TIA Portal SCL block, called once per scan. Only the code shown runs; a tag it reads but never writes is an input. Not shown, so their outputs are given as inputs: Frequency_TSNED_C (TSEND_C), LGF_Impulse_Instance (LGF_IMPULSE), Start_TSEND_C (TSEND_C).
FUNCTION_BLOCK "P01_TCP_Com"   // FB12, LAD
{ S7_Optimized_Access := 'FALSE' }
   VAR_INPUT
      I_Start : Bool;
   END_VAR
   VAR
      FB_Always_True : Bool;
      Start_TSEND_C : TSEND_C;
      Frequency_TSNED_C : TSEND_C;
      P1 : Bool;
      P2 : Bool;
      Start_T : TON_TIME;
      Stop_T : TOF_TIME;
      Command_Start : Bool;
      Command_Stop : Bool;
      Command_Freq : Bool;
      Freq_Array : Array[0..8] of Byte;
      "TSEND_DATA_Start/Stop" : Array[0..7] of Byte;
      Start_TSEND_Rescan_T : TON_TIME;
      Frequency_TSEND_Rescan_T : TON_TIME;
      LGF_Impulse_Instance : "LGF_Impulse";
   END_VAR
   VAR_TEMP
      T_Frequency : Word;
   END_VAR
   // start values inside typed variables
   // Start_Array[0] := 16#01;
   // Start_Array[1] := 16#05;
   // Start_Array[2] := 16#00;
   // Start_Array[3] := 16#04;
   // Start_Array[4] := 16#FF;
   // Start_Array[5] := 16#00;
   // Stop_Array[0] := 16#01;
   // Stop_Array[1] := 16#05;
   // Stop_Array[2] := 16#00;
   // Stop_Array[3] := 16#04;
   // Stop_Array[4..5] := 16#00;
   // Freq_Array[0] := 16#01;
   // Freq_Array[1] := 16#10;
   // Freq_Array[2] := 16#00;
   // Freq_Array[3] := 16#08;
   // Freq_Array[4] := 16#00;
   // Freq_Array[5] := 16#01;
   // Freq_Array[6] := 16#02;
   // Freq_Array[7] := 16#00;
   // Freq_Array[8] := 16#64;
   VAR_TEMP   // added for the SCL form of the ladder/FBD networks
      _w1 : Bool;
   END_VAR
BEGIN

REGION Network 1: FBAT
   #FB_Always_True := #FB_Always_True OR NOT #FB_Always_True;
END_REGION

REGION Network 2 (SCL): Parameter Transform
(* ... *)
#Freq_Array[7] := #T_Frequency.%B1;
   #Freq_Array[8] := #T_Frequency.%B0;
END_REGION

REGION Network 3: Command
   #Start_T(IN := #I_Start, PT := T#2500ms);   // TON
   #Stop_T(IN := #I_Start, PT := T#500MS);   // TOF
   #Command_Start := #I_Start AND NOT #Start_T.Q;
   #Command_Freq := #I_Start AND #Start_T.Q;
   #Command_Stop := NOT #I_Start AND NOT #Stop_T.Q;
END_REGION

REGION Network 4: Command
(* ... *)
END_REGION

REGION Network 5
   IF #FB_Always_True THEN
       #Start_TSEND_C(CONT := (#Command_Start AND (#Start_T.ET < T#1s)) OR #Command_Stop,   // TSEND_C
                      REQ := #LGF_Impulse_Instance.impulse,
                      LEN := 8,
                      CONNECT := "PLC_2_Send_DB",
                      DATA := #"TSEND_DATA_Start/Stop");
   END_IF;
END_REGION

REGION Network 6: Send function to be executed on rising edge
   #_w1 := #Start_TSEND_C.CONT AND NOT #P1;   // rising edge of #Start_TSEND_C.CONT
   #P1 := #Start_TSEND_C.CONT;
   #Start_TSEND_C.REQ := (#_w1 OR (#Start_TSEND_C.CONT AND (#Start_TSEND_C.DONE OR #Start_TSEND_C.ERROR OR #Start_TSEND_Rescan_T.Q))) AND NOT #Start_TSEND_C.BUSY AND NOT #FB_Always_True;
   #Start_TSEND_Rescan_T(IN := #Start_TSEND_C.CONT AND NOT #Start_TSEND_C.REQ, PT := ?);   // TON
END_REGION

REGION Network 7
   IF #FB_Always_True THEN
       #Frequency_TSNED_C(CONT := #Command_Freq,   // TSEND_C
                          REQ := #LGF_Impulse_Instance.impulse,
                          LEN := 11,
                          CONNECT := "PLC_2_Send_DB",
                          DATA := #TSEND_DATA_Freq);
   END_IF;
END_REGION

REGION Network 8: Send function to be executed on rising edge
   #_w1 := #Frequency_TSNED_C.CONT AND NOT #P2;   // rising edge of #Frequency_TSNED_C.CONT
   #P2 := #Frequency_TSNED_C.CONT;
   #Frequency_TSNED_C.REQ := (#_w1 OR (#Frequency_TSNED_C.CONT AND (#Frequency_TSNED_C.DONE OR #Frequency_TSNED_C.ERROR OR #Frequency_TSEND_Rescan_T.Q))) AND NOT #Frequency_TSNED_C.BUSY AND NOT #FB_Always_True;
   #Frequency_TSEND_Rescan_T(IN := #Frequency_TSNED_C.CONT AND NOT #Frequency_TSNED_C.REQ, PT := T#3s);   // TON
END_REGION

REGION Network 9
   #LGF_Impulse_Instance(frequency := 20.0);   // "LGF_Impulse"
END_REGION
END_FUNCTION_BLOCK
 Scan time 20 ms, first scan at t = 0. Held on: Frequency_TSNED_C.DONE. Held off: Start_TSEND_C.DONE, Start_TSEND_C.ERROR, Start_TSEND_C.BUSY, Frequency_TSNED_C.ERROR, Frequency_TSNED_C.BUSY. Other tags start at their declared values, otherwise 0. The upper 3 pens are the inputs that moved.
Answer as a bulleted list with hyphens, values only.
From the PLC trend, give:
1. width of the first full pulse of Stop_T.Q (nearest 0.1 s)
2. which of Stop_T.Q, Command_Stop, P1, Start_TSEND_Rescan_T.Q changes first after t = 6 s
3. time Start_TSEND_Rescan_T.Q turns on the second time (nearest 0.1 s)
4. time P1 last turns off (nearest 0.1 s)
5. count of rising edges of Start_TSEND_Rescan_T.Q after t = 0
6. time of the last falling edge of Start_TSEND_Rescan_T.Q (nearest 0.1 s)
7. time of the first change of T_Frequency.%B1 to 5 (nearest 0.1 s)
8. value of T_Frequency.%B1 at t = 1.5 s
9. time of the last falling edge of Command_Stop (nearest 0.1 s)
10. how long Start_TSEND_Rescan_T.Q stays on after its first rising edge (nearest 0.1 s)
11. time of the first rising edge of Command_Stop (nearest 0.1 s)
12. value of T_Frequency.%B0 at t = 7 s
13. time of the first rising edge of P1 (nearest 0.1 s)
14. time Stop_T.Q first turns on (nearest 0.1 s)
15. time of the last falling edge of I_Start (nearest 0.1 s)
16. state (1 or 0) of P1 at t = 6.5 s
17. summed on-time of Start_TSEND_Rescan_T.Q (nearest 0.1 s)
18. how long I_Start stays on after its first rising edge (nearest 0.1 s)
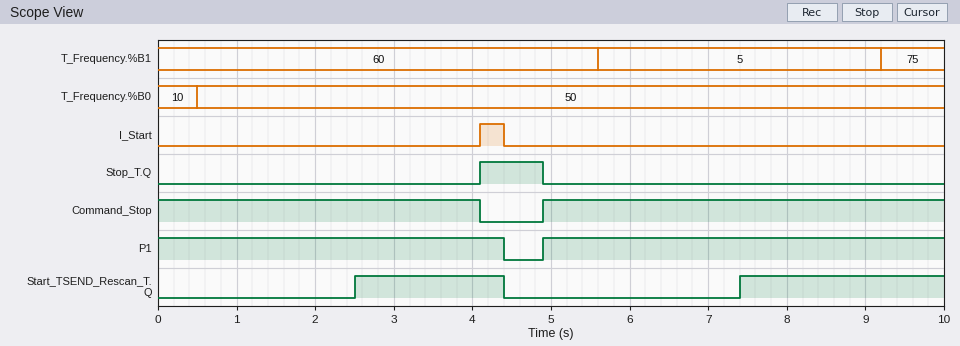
- 0.8 s
- Start_TSEND_Rescan_T.Q
- 7.4 s
- 4.4 s
- 2
- 4.4 s
- 5.6 s
- 60
- 4.1 s
- 1.9 s
- 4.9 s
- 50
- 4.9 s
- 4.1 s
- 4.4 s
- 1
- 4.5 s
- 0.3 s
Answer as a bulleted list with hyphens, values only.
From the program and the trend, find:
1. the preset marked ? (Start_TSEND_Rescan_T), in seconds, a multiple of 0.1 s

- 2.5 s
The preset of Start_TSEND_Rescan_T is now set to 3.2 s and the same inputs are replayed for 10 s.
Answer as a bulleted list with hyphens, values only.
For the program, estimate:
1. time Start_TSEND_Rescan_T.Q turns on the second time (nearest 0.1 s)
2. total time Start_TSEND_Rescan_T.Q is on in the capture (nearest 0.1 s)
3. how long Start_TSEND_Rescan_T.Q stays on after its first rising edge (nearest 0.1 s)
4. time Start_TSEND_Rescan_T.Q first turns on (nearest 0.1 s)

- 8.1 s
- 3.1 s
- 1.2 s
- 3.2 s
